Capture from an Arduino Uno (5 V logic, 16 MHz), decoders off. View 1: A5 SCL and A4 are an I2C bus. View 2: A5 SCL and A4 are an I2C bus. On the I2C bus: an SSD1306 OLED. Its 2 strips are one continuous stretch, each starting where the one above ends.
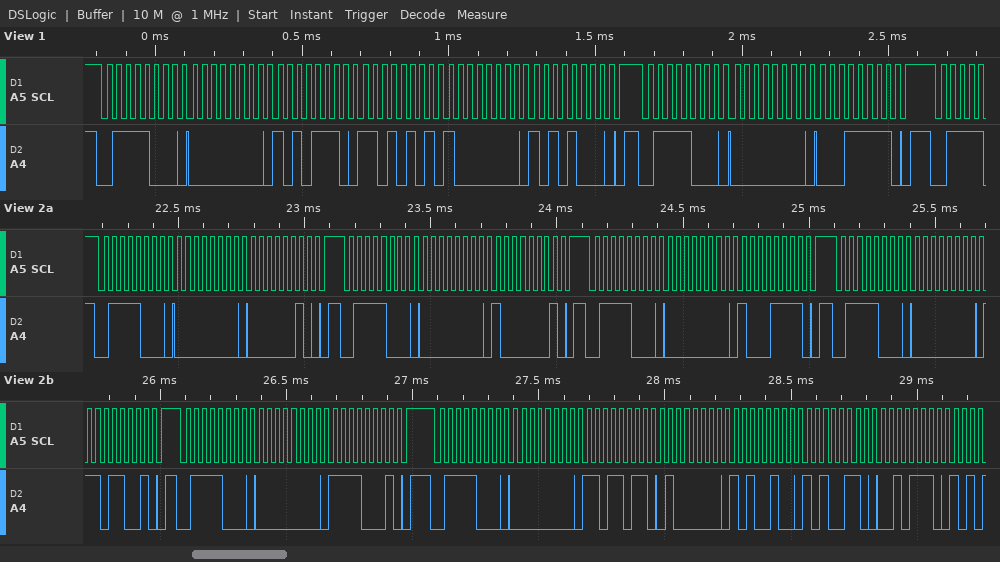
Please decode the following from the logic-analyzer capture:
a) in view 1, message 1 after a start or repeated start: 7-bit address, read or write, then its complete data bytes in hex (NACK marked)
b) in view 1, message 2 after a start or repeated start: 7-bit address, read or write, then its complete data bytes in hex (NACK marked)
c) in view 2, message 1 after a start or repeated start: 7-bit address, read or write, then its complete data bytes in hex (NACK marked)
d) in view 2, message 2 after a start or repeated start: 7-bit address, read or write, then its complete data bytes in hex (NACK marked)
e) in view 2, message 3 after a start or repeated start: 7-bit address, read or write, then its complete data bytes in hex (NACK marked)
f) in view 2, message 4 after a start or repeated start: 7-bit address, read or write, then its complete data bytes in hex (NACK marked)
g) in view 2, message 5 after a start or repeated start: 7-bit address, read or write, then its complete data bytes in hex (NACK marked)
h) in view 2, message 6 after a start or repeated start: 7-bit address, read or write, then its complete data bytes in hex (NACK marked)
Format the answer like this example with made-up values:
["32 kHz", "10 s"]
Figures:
["0x3C write: 00 AE D5 80 A8", "0x3C write: 00 1F", "0x3C write: 00 02", "0x3C write: 00 81", "0x3C write: 00 8F", "0x3C write: 00 D9", "0x3C write: 00 F1", "0x3C write: 00 DB 40 A4 A6 2E"]
